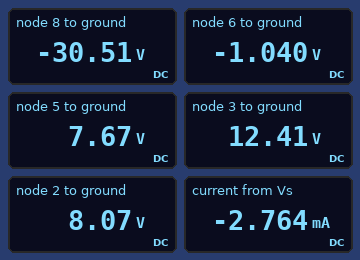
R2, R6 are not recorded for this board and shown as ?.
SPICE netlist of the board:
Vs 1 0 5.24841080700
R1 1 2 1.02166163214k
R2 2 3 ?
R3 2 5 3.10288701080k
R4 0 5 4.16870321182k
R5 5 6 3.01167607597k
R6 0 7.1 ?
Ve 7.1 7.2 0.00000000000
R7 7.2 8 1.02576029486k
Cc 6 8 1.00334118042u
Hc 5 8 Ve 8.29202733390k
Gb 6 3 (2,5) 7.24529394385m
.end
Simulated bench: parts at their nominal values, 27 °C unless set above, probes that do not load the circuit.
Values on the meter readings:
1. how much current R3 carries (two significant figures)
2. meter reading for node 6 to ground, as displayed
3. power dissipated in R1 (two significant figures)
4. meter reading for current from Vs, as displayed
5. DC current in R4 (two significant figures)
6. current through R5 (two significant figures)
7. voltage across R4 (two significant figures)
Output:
130 µA
-1.040 V
7.8 mW
-2.764 mA
1.8 mA
2.9 mA
7.7 V
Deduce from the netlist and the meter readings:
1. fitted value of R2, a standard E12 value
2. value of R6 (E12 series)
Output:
1.5 kΩ
5.6 kΩ
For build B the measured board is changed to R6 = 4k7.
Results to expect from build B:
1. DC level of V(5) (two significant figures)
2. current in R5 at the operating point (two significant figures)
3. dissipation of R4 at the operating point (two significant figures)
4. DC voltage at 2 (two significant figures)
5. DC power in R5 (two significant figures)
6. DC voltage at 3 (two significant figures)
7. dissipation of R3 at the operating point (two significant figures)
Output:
6.0 V
950 µA
8.8 mW
6.2 V
2.7 mW
7.6 V
5.5 µW
